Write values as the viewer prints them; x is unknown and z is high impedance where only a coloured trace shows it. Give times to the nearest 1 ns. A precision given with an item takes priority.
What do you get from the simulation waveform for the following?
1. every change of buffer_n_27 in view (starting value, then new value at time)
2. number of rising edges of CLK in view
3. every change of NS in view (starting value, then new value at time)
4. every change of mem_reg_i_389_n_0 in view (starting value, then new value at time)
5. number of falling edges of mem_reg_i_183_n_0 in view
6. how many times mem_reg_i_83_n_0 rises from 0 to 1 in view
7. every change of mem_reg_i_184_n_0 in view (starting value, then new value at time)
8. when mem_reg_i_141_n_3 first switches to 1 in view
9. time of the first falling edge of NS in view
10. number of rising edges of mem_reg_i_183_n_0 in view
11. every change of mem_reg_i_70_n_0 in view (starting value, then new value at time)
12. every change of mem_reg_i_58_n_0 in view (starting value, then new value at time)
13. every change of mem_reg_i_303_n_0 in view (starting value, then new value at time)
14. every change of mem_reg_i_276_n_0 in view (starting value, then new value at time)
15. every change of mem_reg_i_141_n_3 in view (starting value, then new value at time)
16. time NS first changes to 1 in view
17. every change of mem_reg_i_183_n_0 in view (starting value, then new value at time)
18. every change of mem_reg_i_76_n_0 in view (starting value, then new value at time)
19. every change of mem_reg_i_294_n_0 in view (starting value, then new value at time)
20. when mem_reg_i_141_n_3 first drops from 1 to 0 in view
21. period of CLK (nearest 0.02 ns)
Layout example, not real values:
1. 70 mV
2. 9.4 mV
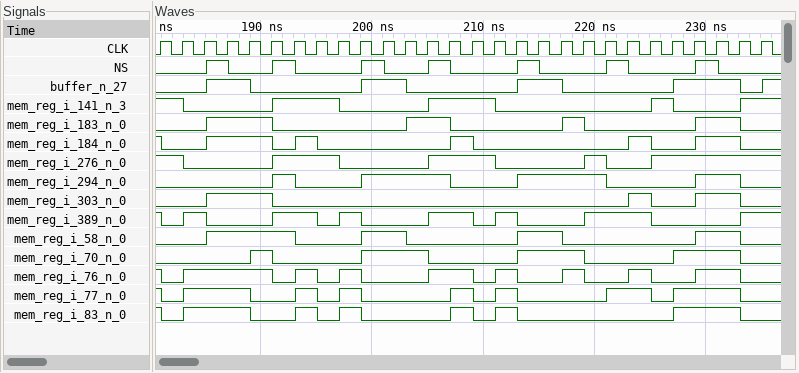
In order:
1. 0, 1 at 185 ns, 0 at 189 ns, 1 at 199 ns, 0 at 203 ns, 1 at 213 ns, 0 at 217 ns, 1 at 227 ns, 0 at 233 ns, 1 at 235 ns
2. 28
3. 0, 1 at 185 ns, 0 at 187 ns, 1 at 191 ns, 0 at 193 ns, 1 at 199 ns, 0 at 201 ns, 1 at 205 ns, 0 at 207 ns, 1 at 213 ns, 0 at 215 ns, 1 at 221 ns, 0 at 223 ns, 1 at 229 ns, 0 at 231 ns
4. 1, 0 at 181 ns, 1 at 183 ns, 0 at 185 ns, 1 at 191 ns, 0 at 195 ns, 1 at 197 ns, 0 at 199 ns, 1 at 205 ns, 0 at 209 ns, 1 at 211 ns, 0 at 213 ns, 1 at 219 ns, 0 at 225 ns, 1 at 233 ns
5. 4
6. 6
7. 1, 0 at 181 ns, 1 at 185 ns, 0 at 191 ns, 1 at 193 ns, 0 at 195 ns, 1 at 207 ns, 0 at 209 ns, 1 at 223 ns, 0 at 225 ns, 1 at 229 ns, 0 at 233 ns
8. 191 ns
9. 187 ns
10. 4
11. 0, 1 at 189 ns, 0 at 191 ns, 1 at 199 ns, 0 at 205 ns, 1 at 213 ns, 0 at 219 ns, 1 at 227 ns, 0 at 233 ns
12. 0, 1 at 185 ns, 0 at 193 ns, 1 at 199 ns, 0 at 203 ns, 1 at 213 ns, 0 at 217 ns, 1 at 229 ns, 0 at 233 ns
13. 0, 1 at 185 ns, 0 at 191 ns, 1 at 223 ns, 0 at 225 ns, 1 at 229 ns, 0 at 233 ns
14. 1, 0 at 183 ns, 1 at 191 ns, 0 at 197 ns, 1 at 205 ns, 0 at 211 ns, 1 at 219 ns, 0 at 221 ns, 1 at 225 ns
15. 1, 0 at 183 ns, 1 at 191 ns, 0 at 197 ns, 1 at 205 ns, 0 at 211 ns, 1 at 225 ns, 0 at 227 ns, 1 at 233 ns
16. 185 ns
17. 0, 1 at 185 ns, 0 at 191 ns, 1 at 203 ns, 0 at 207 ns, 1 at 217 ns, 0 at 219 ns, 1 at 229 ns, 0 at 233 ns
18. 1, 0 at 181 ns, 1 at 183 ns, 0 at 191 ns, 1 at 193 ns, 0 at 195 ns, 1 at 197 ns, 0 at 199 ns, 1 at 205 ns, 0 at 209 ns, 1 at 211 ns, 0 at 213 ns, 1 at 217 ns, 0 at 219 ns, 1 at 223 ns, 0 at 225 ns, 1 at 229 ns, 0 at 233 ns
19. 0, 1 at 191 ns, 0 at 193 ns, 1 at 199 ns, 0 at 207 ns, 1 at 213 ns, 0 at 221 ns, 1 at 229 ns, 0 at 233 ns
20. 183 ns
21. 2 ns
